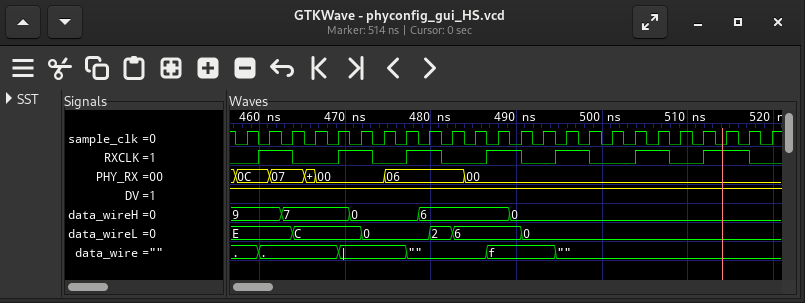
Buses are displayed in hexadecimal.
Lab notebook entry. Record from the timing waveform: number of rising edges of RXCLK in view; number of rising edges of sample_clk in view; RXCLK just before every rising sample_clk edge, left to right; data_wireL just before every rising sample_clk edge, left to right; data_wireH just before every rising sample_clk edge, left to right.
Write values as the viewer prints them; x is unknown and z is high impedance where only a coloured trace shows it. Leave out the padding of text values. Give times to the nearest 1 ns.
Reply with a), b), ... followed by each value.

a) 7
b) 24
c) 0 1 1 0 0 1 0 0 1 0 0 1 1 0 1 1 0 0 1 0 0 1 1 0
d) E, E, E, C, C, C, 0, 0, 0, 2, 6, 6, 6, 0, 0, 0, 0, 0, 0, 0, 0, 0, 0, 0
e) 9, 9, 7, 7, 7, 0, 0, 0, 6, 6, 6, 6, 0, 0, 0, 0, 0, 0, 0, 0, 0, 0, 0, 0
